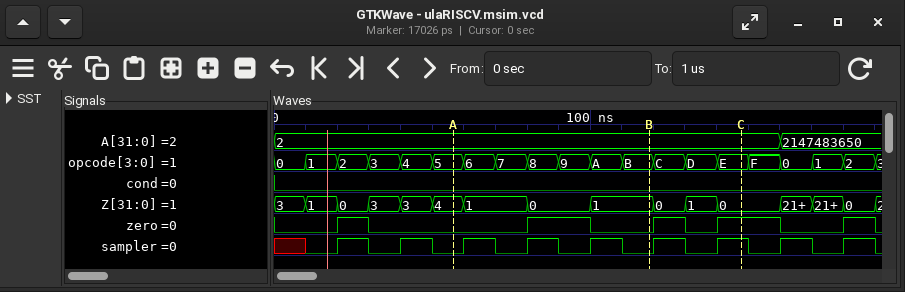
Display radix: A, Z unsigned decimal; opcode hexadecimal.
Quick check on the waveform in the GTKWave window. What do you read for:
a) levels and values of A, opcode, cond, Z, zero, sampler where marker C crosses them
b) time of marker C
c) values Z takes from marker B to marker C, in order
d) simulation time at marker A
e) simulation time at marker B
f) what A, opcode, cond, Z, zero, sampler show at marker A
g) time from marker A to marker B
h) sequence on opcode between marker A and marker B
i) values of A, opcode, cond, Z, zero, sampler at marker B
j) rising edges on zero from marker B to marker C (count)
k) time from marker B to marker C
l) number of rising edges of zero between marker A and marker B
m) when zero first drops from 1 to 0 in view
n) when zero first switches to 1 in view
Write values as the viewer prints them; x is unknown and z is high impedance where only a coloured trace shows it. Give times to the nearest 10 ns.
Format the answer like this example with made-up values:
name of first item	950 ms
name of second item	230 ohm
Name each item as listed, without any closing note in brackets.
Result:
levels and values of A, opcode, cond, Z, zero, sampler where marker C crosses them	A=2, opcode=E, cond=0, Z=0, zero=1, sampler=1
time of marker C	150 ns
values Z takes from marker B to marker C, in order	1, 0, 1, 0
simulation time at marker A	60 ns
simulation time at marker B	120 ns
what A, opcode, cond, Z, zero, sampler show at marker A	A=2, opcode=5, cond=0, Z=4, zero=0, sampler=0
time from marker A to marker B	60 ns
sequence on opcode between marker A and marker B	5, 6, 7, 8, 9, A, B
values of A, opcode, cond, Z, zero, sampler at marker B	A=2, opcode=B, cond=0, Z=1, zero=0, sampler=0
rising edges on zero from marker B to marker C	2
time from marker B to marker C	30 ns
number of rising edges of zero between marker A and marker B	1
when zero first drops from 1 to 0 in view	30 ns
when zero first switches to 1 in view	20 ns
